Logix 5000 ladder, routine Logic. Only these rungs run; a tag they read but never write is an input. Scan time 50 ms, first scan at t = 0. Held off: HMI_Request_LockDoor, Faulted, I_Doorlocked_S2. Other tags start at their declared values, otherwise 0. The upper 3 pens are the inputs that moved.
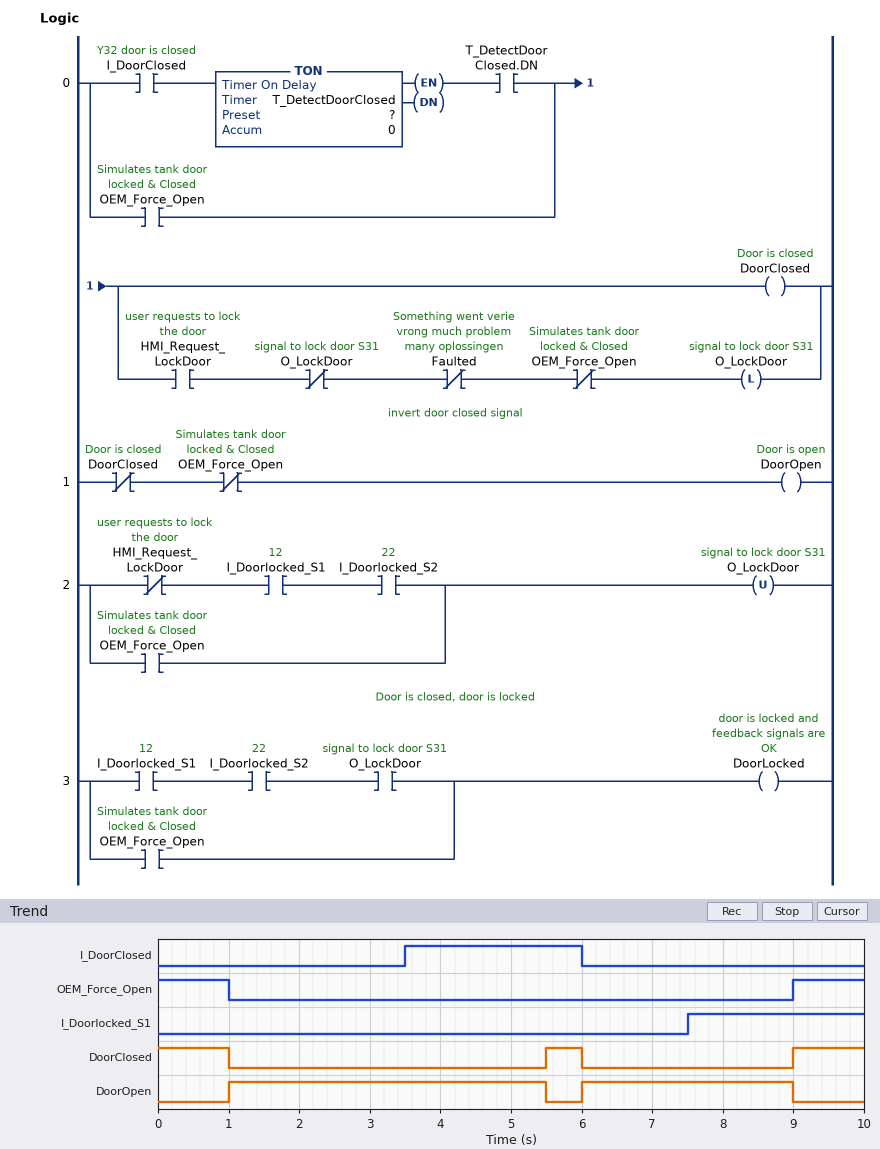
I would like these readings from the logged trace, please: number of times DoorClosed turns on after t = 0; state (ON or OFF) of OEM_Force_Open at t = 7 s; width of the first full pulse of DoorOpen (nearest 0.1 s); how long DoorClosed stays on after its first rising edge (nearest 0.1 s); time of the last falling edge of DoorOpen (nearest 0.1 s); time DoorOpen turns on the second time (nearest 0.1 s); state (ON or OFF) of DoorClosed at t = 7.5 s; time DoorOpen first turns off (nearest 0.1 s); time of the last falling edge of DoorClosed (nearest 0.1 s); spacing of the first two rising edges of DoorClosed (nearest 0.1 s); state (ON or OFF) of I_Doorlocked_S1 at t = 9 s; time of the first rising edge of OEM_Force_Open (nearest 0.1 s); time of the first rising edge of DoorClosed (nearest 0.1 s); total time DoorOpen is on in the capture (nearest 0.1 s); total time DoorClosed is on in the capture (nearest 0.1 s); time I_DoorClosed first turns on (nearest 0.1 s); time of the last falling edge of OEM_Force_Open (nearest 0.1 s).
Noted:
2
OFF
4.5 s
0.5 s
9.0 s
6.0 s
OFF
5.5 s
6.0 s
3.5 s
ON
9.0 s
5.5 s
7.5 s
2.5 s
3.5 s
1.0 s
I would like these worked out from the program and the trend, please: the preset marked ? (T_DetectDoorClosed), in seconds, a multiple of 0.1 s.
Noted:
2.0 s
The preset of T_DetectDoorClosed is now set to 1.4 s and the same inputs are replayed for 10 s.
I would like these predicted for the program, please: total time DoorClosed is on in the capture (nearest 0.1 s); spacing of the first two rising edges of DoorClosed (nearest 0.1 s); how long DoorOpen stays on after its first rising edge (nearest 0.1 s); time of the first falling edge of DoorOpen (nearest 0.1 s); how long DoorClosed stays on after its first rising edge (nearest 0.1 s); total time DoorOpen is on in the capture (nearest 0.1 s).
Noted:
3.1 s
4.1 s
3.9 s
4.9 s
1.1 s
6.9 s
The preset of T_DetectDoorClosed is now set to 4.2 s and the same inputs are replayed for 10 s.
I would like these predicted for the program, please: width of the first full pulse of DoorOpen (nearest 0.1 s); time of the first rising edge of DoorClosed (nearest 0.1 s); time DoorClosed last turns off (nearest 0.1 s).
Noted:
8.0 s
9.0 s
1.0 s
